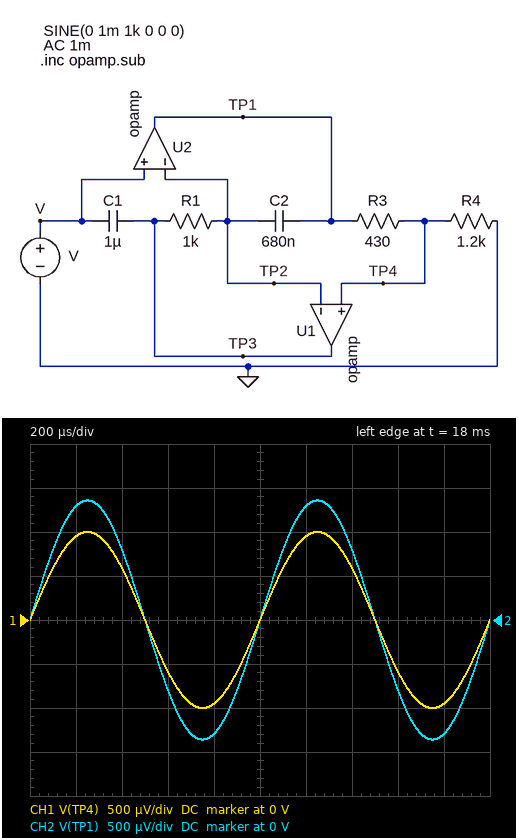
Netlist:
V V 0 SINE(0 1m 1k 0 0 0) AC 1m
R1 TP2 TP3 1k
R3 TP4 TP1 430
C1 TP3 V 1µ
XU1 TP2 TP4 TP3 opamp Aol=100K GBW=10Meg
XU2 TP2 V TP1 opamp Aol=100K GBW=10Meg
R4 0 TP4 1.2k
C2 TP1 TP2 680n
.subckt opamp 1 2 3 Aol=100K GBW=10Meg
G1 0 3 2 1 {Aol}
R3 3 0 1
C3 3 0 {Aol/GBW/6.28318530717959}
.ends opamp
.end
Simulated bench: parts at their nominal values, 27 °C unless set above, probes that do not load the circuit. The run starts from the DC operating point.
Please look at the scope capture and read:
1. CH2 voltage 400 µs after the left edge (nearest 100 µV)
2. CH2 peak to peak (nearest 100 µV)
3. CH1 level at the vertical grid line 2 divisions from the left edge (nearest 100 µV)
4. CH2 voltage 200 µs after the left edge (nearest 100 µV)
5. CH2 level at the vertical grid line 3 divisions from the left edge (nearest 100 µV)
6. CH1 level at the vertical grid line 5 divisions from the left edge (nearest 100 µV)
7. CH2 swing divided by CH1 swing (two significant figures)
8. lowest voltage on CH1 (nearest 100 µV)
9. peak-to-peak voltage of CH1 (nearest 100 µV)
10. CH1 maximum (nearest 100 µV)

800 µV
2.7 mV
600 µV
1.3 mV
-800 µV
0 V
1.4
-1.0 mV
2.0 mV
1.0 mV
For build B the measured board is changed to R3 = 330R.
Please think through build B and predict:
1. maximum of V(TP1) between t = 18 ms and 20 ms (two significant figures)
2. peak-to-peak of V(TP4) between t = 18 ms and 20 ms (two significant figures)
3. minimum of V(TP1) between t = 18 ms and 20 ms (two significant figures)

1.3 mV
2.0 mV
-1.3 mV
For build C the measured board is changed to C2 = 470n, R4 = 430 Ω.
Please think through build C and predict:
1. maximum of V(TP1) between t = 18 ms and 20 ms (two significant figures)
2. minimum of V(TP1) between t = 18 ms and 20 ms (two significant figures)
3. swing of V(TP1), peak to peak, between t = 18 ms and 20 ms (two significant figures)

2.0 mV
-2.0 mV
4.0 mV
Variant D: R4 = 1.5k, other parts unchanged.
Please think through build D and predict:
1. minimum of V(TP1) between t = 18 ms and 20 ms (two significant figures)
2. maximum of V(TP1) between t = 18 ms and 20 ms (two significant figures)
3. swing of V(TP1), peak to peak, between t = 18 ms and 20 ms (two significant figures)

-1.3 mV
1.3 mV
2.6 mV
